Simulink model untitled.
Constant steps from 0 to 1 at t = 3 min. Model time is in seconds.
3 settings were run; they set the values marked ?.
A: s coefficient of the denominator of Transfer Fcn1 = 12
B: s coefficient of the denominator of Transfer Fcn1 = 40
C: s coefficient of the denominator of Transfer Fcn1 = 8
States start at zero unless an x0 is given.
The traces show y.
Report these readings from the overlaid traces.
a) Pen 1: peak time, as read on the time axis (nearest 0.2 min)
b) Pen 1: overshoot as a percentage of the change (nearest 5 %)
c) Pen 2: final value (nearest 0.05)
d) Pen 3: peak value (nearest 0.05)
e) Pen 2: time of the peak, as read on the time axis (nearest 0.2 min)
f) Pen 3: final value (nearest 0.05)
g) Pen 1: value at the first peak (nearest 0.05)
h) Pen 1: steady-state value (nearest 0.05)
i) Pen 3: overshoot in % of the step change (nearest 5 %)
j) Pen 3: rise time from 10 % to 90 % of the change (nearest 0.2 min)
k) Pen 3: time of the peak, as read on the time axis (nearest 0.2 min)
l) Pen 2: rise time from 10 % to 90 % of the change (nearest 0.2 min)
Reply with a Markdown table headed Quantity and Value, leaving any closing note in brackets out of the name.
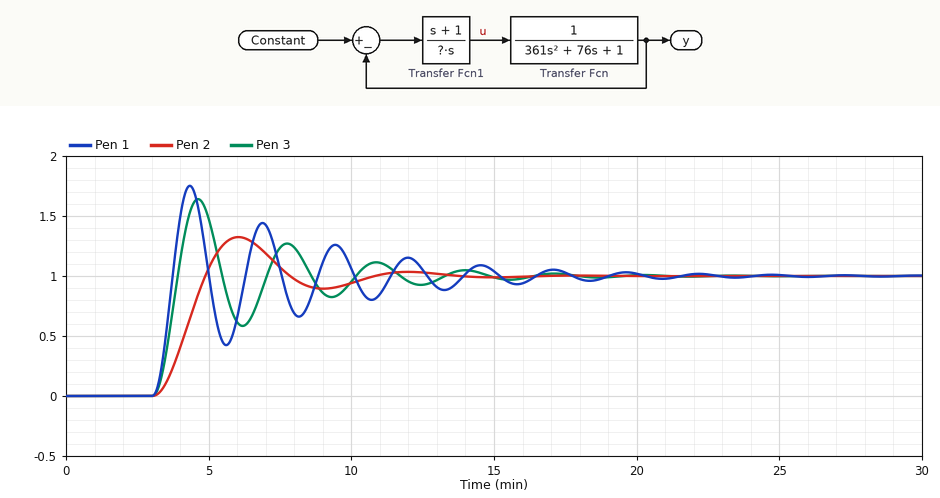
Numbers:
| Quantity | Value |
|---|---|
| Pen 1: peak time, as read on the time axis | 4.4 min |
| Pen 1: overshoot as a percentage of the change | 75 % |
| Pen 2: final value | 1.00 |
| Pen 3: peak value | 1.65 |
| Pen 2: time of the peak, as read on the time axis | 6.0 min |
| Pen 3: final value | 1.00 |
| Pen 1: value at the first peak | 1.75 |
| Pen 1: steady-state value | 1.00 |
| Pen 3: overshoot in % of the step change | 65 % |
| Pen 3: rise time from 10 % to 90 % of the change | 0.6 min |
| Pen 3: time of the peak, as read on the time axis | 4.6 min |
| Pen 2: rise time from 10 % to 90 % of the change | 1.2 min |
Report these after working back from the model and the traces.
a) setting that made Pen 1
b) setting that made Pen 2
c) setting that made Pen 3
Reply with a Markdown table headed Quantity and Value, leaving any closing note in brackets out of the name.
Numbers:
| Quantity | Value |
|---|---|
| setting that made Pen 1 | C |
| setting that made Pen 2 | B |
| setting that made Pen 3 | A |
